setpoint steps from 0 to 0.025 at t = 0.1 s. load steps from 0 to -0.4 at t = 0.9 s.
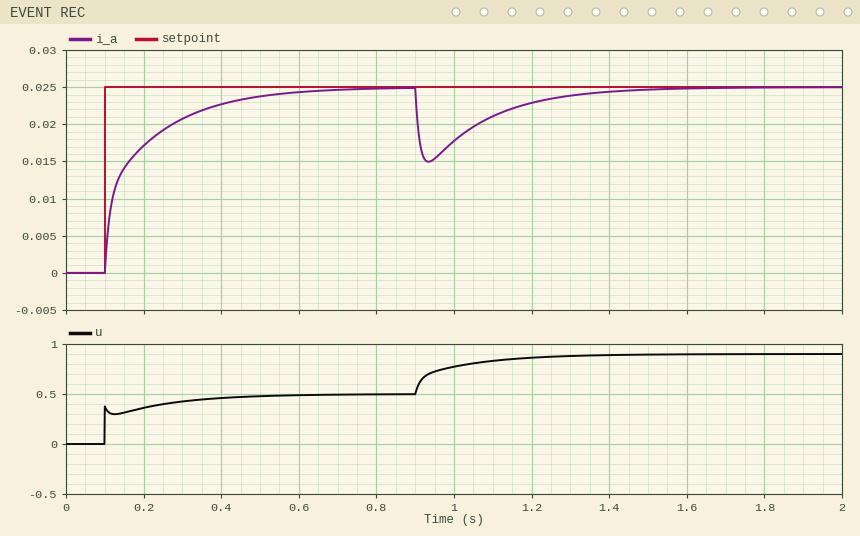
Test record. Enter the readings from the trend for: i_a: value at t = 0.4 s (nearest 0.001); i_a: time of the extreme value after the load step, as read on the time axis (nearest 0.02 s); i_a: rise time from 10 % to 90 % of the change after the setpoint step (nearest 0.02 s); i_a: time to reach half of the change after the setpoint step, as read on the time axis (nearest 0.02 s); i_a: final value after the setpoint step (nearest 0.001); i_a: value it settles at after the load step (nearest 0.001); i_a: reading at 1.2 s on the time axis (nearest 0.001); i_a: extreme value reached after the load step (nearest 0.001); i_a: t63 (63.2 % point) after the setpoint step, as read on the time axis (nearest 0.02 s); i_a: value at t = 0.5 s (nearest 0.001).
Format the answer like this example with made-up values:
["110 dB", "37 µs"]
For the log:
["0.023", "0.94 s", "0.28 s", "0.14 s", "0.025", "0.025", "0.023", "0.015", "0.18 s", "0.024"]
